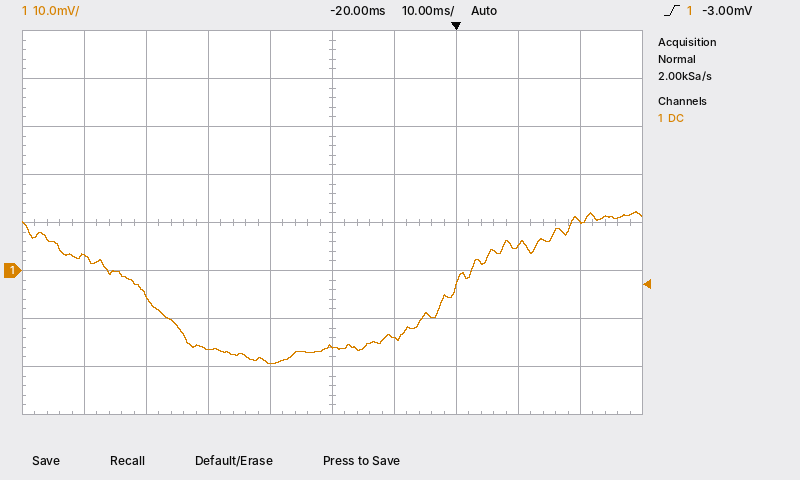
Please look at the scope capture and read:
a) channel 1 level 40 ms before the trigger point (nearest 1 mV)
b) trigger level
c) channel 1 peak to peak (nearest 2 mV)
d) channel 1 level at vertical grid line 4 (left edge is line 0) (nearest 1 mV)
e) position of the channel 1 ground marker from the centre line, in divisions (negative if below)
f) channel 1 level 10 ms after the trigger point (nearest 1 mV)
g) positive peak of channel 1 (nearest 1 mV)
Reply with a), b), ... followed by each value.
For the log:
a) -16 mV
b) -3.00 mV
c) 32 mV
d) -19 mV
e) -1.0 div
f) 5 mV
g) 12 mV
